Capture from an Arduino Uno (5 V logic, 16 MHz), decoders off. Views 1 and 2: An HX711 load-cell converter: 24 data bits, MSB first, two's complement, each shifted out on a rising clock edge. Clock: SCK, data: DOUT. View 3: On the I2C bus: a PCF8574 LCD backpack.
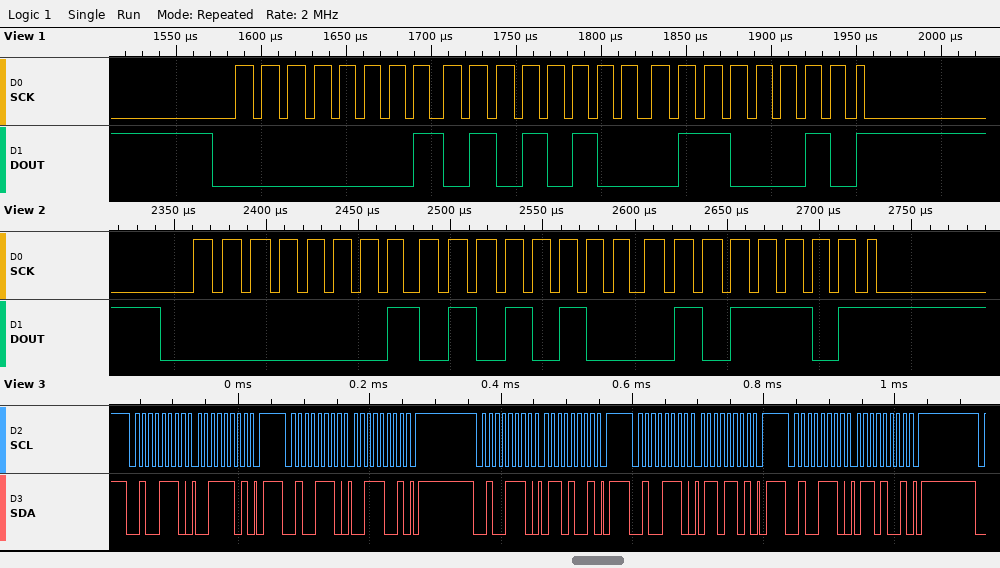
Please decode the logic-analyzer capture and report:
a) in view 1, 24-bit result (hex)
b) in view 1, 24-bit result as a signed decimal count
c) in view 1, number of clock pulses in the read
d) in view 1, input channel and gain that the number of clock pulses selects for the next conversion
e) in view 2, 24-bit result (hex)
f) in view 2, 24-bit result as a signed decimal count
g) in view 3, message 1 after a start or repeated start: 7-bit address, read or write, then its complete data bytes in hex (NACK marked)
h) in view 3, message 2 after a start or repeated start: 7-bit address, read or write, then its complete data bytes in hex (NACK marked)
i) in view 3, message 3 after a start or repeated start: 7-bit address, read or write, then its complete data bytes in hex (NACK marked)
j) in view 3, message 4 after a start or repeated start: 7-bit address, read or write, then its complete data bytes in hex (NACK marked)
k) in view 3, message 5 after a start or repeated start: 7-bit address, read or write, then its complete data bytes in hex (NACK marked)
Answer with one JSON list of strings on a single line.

["0x015462", "87138", "25", "channel A, gain 128", "0x01545D", "87133", "0x27 write: 3D", "0x27 write: 39", "0x27 write: 69", "0x27 write: 6D", "0x27 write: 69"]
